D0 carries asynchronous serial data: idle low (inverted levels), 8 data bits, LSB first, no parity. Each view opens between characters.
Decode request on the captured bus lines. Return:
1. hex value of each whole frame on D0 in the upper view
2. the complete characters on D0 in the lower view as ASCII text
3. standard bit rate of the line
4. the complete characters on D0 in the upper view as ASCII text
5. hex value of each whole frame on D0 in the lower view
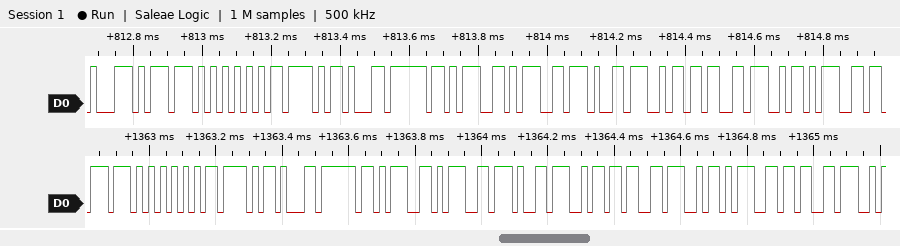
47, 44, 55, 42, 3A, 20, 31, 31, 34, 2C, 32, 2C, 31
"DUB: 114,2,12"
57600 baud
"GDUB: 114,2,1"
44, 55, 42, 3A, 20, 31, 31, 34, 2C, 32, 2C, 31, 32
